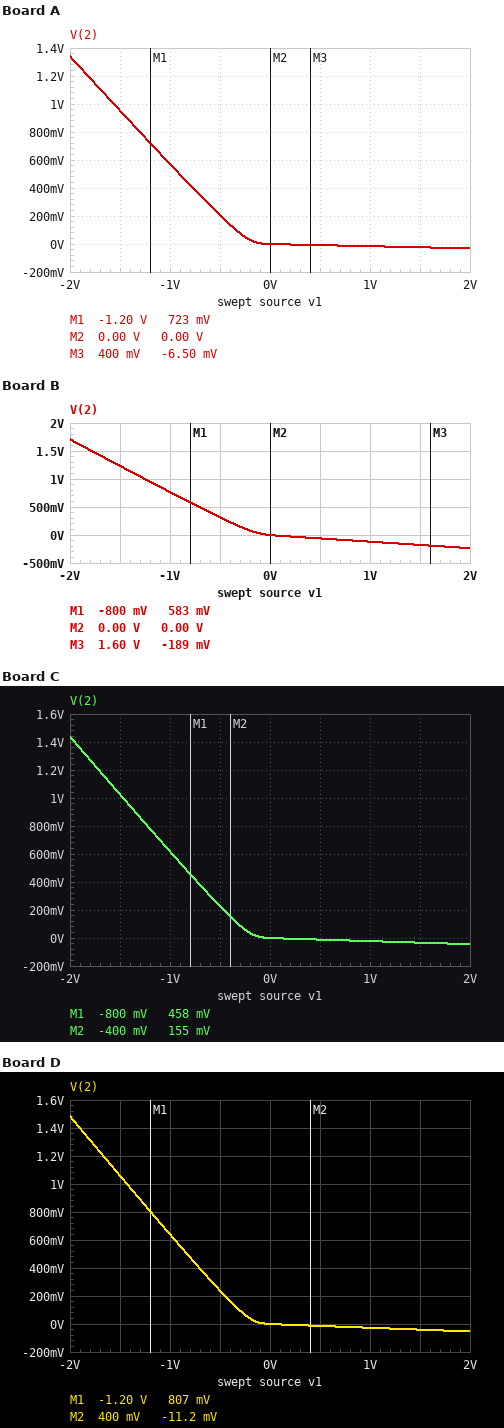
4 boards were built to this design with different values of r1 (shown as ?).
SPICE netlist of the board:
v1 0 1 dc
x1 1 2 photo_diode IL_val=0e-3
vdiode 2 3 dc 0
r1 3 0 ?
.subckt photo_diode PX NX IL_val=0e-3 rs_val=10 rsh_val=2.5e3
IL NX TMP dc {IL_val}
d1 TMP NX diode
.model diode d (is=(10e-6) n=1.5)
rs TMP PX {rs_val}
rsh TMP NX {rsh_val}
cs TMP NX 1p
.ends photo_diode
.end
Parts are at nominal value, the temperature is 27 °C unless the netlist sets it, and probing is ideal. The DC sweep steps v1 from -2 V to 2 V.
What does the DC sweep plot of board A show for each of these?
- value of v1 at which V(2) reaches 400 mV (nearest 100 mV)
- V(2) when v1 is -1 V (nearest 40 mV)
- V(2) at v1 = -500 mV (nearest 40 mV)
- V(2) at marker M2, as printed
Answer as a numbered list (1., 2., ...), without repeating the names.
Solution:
1. -800 mV
2. 560 mV
3. 200 mV
4. 0.00 V
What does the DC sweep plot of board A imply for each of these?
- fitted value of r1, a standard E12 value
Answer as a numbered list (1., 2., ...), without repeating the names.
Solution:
1. 39 Ω
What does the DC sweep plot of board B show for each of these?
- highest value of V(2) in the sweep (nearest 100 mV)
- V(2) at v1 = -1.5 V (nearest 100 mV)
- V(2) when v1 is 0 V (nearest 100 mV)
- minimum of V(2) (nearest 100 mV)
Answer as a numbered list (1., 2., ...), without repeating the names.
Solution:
1. 1.7 V
2. 1.2 V
3. 0 V
4. -200 mV
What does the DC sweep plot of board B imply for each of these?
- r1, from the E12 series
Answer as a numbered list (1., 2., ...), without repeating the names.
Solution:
1. 330 Ω
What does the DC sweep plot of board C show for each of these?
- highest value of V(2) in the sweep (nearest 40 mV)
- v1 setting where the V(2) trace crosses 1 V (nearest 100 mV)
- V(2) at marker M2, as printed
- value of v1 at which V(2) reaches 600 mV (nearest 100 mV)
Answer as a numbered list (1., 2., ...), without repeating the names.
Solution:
1. 1.44 V
2. -1.5 V
3. 155 mV
4. -1.0 V
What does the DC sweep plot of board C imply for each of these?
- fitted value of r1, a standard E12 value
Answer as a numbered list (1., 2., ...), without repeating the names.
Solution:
1. 56 Ω
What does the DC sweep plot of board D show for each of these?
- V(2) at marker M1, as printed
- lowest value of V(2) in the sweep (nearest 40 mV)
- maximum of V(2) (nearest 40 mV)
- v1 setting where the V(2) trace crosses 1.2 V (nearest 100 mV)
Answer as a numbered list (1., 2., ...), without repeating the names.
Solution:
1. 807 mV
2. -40 mV
3. 1.48 V
4. -1.7 V
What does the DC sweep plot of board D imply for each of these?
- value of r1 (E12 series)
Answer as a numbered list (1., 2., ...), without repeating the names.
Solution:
1. 68 Ω
